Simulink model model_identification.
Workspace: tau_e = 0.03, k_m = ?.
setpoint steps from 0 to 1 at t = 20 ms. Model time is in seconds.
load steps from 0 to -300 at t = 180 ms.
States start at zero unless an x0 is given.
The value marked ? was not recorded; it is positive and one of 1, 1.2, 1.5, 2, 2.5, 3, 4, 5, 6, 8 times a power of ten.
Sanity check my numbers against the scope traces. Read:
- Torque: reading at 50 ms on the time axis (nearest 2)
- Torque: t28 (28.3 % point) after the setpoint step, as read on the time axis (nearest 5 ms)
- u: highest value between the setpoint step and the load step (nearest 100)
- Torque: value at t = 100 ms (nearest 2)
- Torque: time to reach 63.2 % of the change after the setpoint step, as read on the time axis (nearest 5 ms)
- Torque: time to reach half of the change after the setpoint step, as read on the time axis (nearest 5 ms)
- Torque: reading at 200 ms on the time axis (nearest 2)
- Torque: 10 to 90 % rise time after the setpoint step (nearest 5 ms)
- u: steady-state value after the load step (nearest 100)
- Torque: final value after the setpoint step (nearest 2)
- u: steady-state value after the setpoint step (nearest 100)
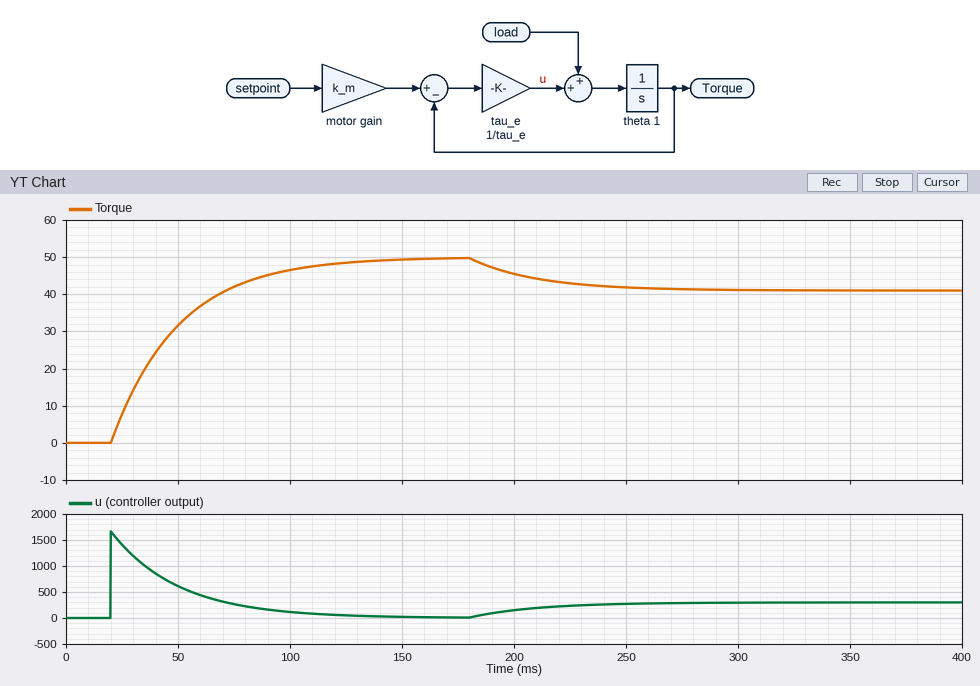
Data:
32
30 ms
1700
46
50 ms
40 ms
46
65 ms
300
50
0
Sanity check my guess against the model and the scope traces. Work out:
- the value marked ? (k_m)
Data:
50
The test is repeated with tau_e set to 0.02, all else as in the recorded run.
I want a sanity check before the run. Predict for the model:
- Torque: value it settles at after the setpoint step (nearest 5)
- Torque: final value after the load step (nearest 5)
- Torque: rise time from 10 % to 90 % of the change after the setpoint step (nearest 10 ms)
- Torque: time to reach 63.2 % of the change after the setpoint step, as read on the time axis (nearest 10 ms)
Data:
50
45
40 ms
40 ms
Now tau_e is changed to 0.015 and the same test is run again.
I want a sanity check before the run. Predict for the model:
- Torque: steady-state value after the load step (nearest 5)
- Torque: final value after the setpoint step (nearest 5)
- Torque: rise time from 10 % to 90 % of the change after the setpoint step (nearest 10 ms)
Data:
45
50
30 ms
